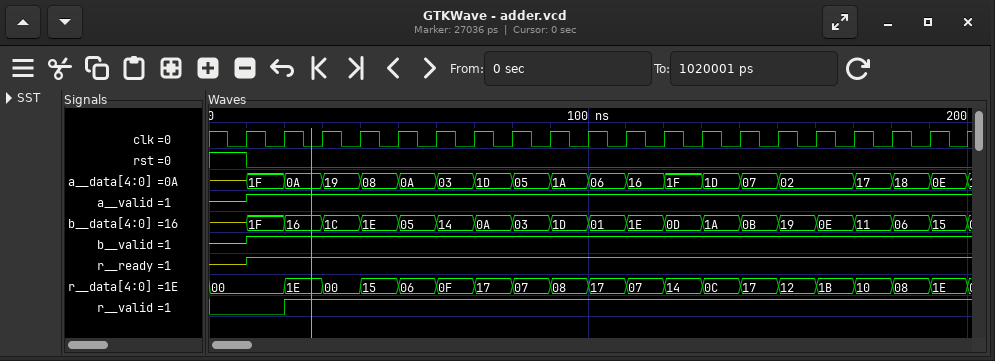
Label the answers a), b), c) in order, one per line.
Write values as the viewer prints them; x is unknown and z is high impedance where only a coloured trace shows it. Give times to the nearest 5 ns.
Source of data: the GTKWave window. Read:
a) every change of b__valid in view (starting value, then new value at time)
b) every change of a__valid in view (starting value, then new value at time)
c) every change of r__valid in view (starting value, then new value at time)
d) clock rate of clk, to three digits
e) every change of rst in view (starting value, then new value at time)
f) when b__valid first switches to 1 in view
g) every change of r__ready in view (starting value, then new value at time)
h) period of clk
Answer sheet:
a) z, 1 at 10 ns
b) z, 1 at 10 ns
c) 0, 1 at 20 ns
d) 100 MHz
e) 1, 0 at 10 ns
f) 10 ns
g) z, 1 at 10 ns
h) 10 ns
